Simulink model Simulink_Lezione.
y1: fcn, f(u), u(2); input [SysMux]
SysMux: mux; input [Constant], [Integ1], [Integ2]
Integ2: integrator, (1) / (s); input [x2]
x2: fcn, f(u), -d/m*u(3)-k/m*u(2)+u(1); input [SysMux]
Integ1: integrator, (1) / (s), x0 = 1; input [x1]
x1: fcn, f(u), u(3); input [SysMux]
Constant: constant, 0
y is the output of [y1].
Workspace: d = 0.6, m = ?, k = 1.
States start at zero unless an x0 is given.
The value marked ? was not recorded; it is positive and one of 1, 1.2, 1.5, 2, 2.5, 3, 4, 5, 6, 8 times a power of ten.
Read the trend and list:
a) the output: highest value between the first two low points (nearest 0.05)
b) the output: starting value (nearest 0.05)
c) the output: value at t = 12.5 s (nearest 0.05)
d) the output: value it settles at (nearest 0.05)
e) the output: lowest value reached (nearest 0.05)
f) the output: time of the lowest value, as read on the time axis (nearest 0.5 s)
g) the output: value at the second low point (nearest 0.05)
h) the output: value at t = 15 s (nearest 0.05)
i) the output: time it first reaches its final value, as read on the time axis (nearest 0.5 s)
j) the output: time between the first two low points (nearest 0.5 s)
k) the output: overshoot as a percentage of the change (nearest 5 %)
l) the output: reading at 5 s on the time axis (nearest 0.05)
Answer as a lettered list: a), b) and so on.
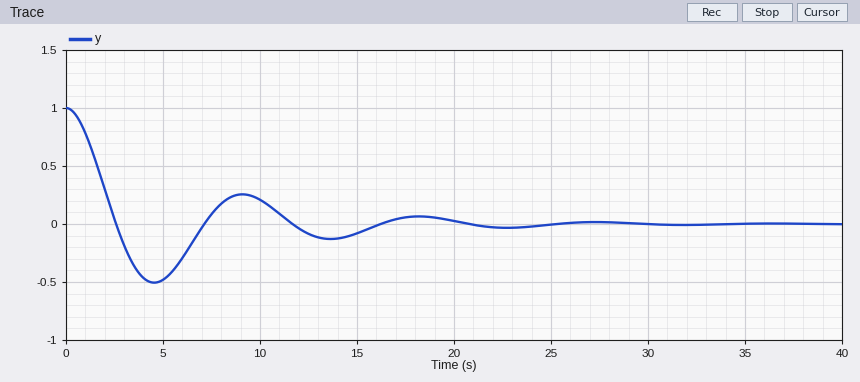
a) 0.25
b) 1.00
c) -0.10
d) 0.00
e) -0.50
f) 4.5 s
g) -0.15
h) -0.10
i) 2.5 s
j) 9.0 s
k) 50 %
l) -0.50
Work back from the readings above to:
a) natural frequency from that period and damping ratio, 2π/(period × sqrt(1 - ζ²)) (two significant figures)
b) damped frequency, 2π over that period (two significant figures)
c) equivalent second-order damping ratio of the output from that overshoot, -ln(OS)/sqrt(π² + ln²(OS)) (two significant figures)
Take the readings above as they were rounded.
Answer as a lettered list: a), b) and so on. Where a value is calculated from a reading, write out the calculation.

a) 2π / (9 × sqrt(1 - 0.22²)) = 0.72 rad/s
b) 2π / 9 = 0.70 rad/s
c) ln(0.5) = -0.693; 0.693 / sqrt(9.870 + 0.480) = 0.22
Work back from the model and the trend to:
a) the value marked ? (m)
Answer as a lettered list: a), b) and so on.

a) 2
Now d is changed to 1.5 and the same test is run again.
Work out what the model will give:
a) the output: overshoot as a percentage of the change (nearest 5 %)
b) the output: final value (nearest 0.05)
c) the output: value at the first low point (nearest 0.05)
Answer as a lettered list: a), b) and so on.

a) 15 %
b) 0.00
c) -0.15
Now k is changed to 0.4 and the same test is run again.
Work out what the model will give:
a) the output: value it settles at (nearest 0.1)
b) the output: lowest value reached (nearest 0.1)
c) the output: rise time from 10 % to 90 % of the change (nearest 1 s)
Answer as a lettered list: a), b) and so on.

a) 0.0
b) -0.3
c) 3 s
